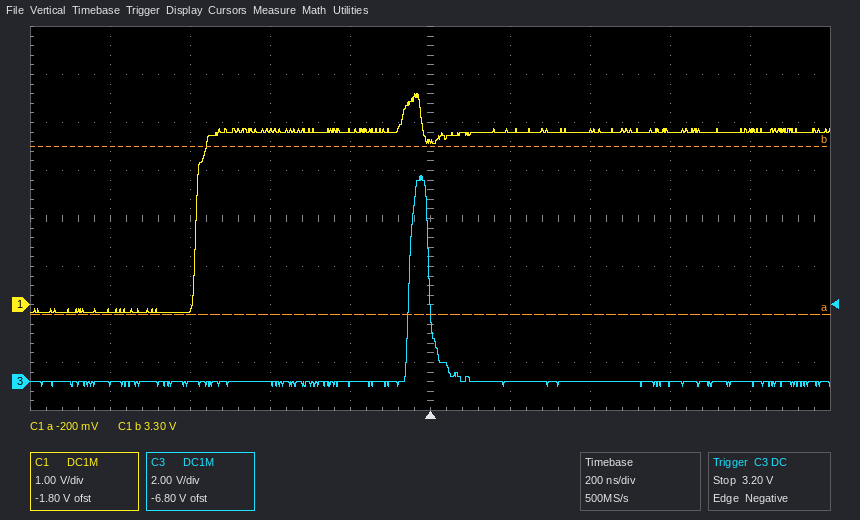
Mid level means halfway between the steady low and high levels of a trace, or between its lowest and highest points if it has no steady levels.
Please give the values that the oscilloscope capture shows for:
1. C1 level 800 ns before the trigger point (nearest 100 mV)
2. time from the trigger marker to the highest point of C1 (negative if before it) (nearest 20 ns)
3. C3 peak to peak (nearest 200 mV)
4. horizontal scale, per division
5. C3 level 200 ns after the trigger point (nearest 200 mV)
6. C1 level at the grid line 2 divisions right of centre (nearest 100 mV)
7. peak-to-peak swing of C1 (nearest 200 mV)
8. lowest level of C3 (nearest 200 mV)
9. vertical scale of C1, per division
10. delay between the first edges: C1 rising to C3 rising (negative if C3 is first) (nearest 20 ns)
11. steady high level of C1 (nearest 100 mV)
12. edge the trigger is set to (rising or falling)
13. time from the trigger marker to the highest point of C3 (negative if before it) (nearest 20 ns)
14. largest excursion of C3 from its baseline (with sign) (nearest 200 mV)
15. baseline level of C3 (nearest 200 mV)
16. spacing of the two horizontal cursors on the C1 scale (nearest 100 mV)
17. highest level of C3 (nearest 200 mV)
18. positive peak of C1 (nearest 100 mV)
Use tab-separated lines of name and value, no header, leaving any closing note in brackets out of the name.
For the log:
C1 level 800 ns before the trigger point	-100 mV
time from the trigger marker to the highest point of C1 (negative if before it)	-40 ns
C3 peak to peak	8.8 V
horizontal scale, per division	200 ns
C3 level 200 ns after the trigger point	0.0 V
C1 level at the grid line 2 divisions right of centre	3.6 V
peak-to-peak swing of C1	4.6 V
lowest level of C3	-200 mV
vertical scale of C1, per division	1 V
delay between the first edges: C1 rising to C3 rising (negative if C3 is first)	+540 ns
steady high level of C1	3.6 V
edge the trigger is set to	falling
time from the trigger marker to the highest point of C3 (negative if before it)	-20 ns
largest excursion of C3 from its baseline (with sign)	+8.6 V
baseline level of C3	0.0 V
spacing of the two horizontal cursors on the C1 scale	3.5 V
highest level of C3	8.6 V
positive peak of C1	4.4 V
